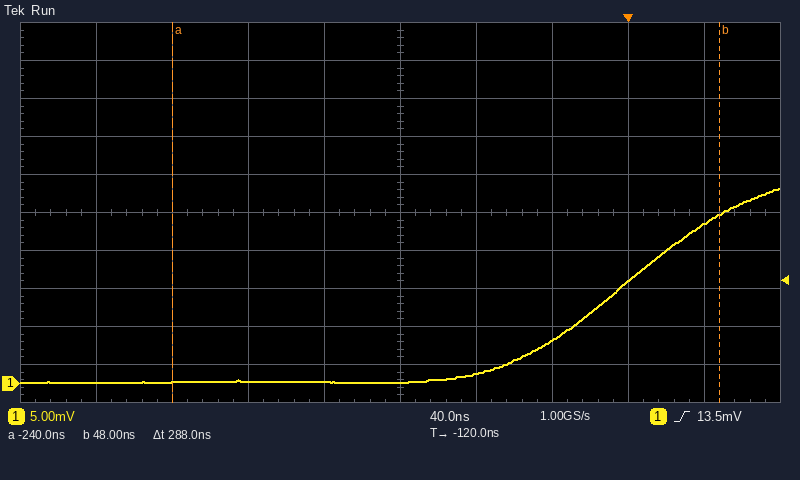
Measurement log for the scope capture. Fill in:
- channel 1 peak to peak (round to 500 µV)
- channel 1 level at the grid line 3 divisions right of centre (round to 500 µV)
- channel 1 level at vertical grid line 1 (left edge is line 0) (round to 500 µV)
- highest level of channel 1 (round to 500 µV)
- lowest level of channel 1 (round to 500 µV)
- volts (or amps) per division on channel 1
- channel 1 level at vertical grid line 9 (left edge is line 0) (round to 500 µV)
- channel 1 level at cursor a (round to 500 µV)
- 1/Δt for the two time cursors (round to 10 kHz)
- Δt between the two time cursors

25.5 mV
13.5 mV
0.0 mV
25.5 mV
0.0 mV
5 mV
21.0 mV
0.0 mV
3.47 MHz
288 ns
